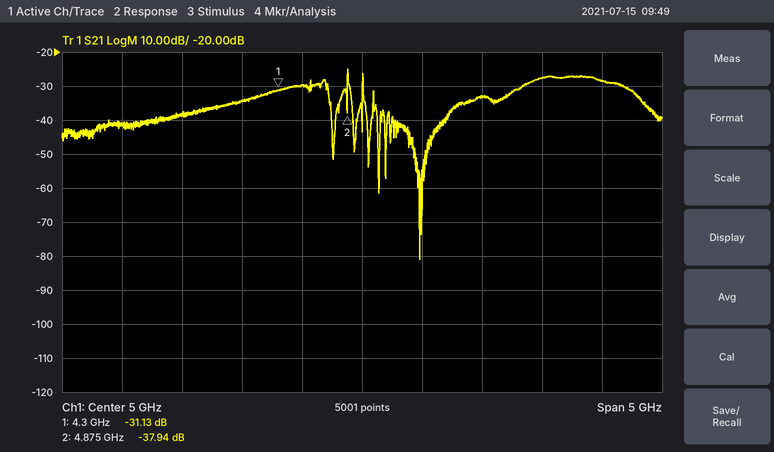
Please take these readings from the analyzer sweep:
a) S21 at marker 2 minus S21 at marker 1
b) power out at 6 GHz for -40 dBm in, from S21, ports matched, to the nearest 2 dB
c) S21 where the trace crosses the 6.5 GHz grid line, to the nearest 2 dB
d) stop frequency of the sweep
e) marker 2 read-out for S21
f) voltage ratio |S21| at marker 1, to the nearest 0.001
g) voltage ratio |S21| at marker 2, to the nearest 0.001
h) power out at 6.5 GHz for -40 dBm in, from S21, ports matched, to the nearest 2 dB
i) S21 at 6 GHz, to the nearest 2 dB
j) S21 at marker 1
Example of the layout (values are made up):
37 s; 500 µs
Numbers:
-6.81 dB; -74 dBm; -28 dB; 7.5 GHz; -37.94 dB; 0.028; 0.013; -68 dBm; -34 dB; -31.13 dB
